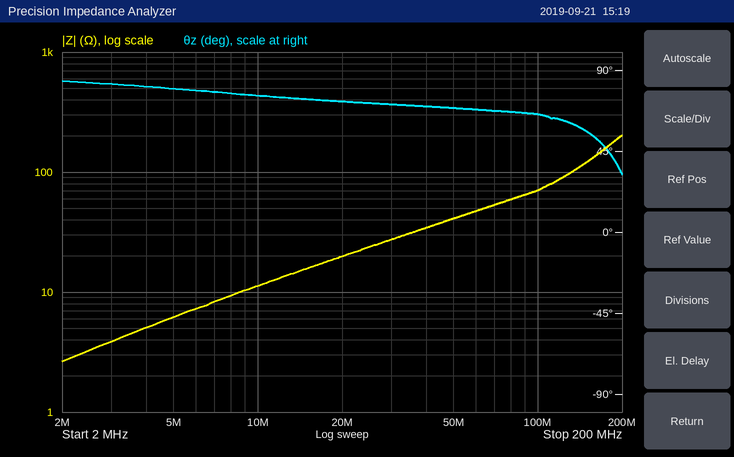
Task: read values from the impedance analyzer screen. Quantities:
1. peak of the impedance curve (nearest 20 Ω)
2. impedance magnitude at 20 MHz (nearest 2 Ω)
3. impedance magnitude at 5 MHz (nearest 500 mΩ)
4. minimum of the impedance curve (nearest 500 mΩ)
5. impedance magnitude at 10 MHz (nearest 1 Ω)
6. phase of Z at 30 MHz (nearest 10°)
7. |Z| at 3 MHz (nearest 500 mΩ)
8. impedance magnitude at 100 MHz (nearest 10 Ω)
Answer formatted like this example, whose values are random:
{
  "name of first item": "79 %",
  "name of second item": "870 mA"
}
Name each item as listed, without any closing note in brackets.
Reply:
{
  "peak of the impedance curve": "200 Ω",
  "impedance magnitude at 20 MHz": "20 Ω",
  "impedance magnitude at 5 MHz": "6.0 Ω",
  "minimum of the impedance curve": "2.5 Ω",
  "impedance magnitude at 10 MHz": "11 Ω",
  "phase of Z at 30 MHz": "70°",
  "|Z| at 3 MHz": "4.0 Ω",
  "impedance magnitude at 100 MHz": "70 Ω"
}
